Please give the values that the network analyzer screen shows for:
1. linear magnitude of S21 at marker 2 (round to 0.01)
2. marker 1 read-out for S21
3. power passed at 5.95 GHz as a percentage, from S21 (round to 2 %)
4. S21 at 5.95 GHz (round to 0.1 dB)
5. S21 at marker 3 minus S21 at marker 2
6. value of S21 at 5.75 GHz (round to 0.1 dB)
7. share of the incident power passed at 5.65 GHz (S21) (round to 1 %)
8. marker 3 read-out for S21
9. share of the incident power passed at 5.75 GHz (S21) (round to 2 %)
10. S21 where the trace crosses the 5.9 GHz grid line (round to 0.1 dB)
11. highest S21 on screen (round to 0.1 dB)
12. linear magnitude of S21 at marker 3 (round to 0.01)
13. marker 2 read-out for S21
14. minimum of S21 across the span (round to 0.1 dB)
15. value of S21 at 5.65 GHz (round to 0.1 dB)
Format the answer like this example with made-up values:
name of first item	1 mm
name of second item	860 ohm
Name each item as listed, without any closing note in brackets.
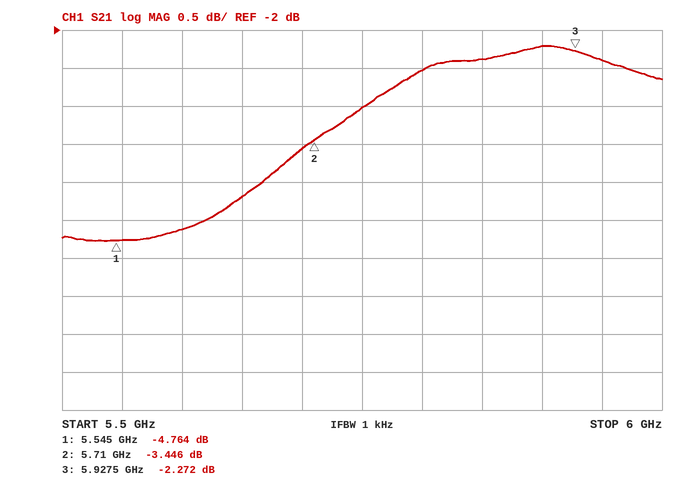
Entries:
linear magnitude of S21 at marker 2	0.67
marker 1 read-out for S21	-4.764 dB
power passed at 5.95 GHz as a percentage, from S21	58 %
S21 at 5.95 GHz	-2.4 dB
S21 at marker 3 minus S21 at marker 2	1.174 dB
value of S21 at 5.75 GHz	-3.0 dB
share of the incident power passed at 5.65 GHz (S21)	38 %
marker 3 read-out for S21	-2.272 dB
share of the incident power passed at 5.75 GHz (S21)	50 %
S21 where the trace crosses the 5.9 GHz grid line	-2.2 dB
highest S21 on screen	-2.2 dB
linear magnitude of S21 at marker 3	0.77
marker 2 read-out for S21	-3.446 dB
minimum of S21 across the span	-4.8 dB
value of S21 at 5.65 GHz	-4.2 dB
